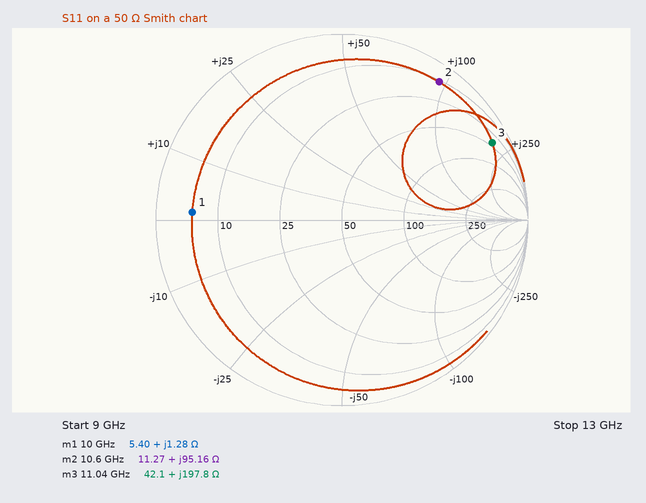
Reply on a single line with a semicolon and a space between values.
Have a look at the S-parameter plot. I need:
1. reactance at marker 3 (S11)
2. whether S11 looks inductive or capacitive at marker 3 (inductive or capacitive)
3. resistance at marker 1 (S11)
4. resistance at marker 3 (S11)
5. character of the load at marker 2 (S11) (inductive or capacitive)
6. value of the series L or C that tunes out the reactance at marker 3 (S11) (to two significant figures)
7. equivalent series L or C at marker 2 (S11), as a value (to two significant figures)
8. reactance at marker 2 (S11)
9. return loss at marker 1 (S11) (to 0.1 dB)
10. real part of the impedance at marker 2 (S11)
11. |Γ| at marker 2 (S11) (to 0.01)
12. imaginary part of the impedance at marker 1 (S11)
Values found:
+197.8 Ω; inductive; 5.40 Ω; 42.1 Ω; inductive; 73 fF; 1.4 nH; +95.16 Ω; 1.9 dB; 11.27 Ω; 0.91; +1.28 Ω
